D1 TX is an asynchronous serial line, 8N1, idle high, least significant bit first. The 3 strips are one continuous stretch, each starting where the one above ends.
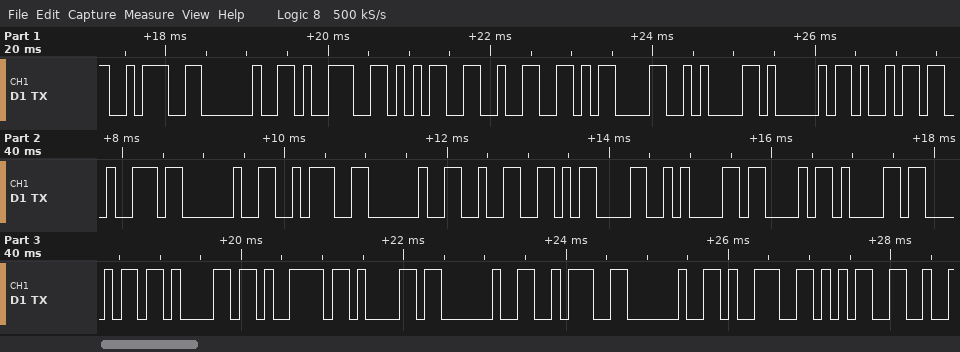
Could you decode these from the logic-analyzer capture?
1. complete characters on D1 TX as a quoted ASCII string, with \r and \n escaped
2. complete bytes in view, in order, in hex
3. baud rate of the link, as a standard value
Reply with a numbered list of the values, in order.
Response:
1. ": 952\r\nAir : 2\r\nCahaya : 95"
2. 3A 20 39 35 32 0D 0A 41 69 72 20 3A 20 32 0D 0A 43 61 68 61 79 61 20 3A 20 39 35
3. 9600 baud
